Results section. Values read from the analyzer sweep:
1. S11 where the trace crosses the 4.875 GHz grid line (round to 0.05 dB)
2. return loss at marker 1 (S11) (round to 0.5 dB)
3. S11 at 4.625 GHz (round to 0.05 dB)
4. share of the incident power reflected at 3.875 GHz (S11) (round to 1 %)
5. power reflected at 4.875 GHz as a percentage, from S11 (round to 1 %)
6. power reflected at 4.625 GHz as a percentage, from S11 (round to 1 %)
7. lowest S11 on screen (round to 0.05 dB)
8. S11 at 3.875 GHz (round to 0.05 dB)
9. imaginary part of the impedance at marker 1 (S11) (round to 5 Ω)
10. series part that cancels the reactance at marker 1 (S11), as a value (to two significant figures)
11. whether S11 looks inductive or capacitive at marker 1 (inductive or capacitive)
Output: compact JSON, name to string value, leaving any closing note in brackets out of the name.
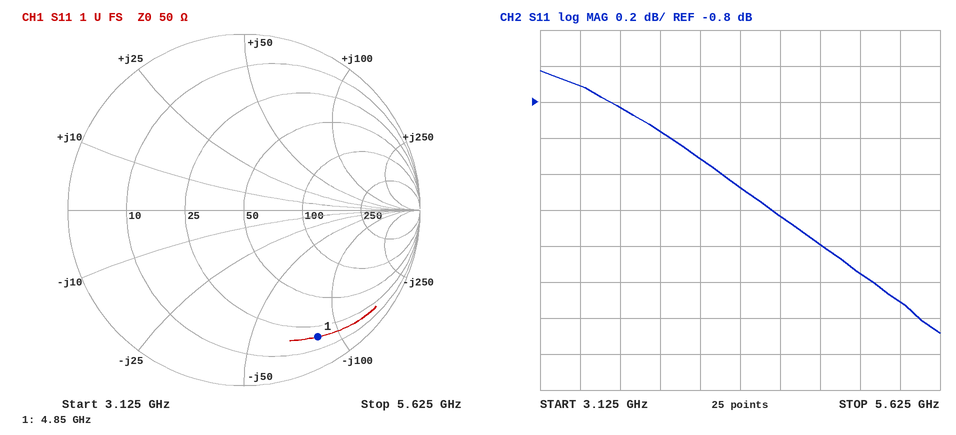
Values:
{"S11 where the trace crosses the 4.875 GHz grid line": "-1.60 dB", "return loss at marker 1 (S11)": "1.5 dB", "S11 at 4.625 GHz": "-1.45 dB", "share of the incident power reflected at 3.875 GHz (S11)": "80 %", "power reflected at 4.875 GHz as a percentage, from S11": "69 %", "power reflected at 4.625 GHz as a percentage, from S11": "72 %", "lowest S11 on screen": "-2.10 dB", "S11 at 3.875 GHz": "-0.95 dB", "imaginary part of the impedance at marker 1 (S11)": "-85 Ω", "series part that cancels the reactance at marker 1 (S11), as a value": "2.8 nH", "whether S11 looks inductive or capacitive at marker 1": "capacitive"}
